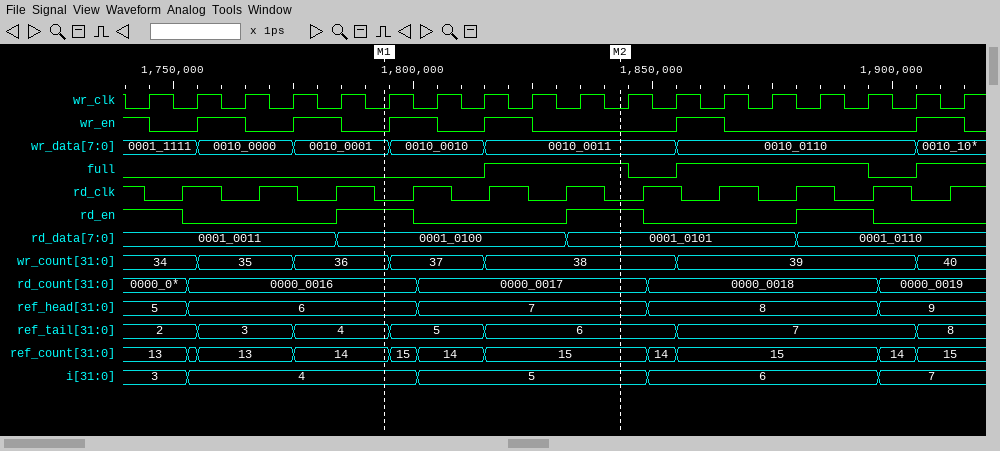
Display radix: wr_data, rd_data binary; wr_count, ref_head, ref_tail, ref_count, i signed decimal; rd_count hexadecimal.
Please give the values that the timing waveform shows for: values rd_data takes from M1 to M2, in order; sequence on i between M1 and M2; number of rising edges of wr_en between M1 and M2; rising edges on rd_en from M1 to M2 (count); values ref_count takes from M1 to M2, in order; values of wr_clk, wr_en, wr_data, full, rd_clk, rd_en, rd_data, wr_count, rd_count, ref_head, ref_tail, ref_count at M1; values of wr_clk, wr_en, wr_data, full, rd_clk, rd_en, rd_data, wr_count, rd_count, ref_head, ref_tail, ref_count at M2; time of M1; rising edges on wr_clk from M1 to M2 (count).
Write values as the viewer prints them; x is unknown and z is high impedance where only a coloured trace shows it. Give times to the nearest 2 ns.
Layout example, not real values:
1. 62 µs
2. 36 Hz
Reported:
1. 0001_0100, 0001_0101
2. 4, 5
3. 2
4. 1
5. 14, 15, 14, 15
6. wr_clk=0, wr_en=0, wr_data=0010_0001, full=0, rd_clk=0, rd_en=1, rd_data=0001_0100, wr_count=36, rd_count=0000_0016, ref_head=6, ref_tail=4, ref_count=14
7. wr_clk=0, wr_en=0, wr_data=0010_0011, full=1, rd_clk=0, rd_en=1, rd_data=0001_0101, wr_count=38, rd_count=0000_0017, ref_head=7, ref_tail=6, ref_count=15
8. 1794 ns
9. 5
